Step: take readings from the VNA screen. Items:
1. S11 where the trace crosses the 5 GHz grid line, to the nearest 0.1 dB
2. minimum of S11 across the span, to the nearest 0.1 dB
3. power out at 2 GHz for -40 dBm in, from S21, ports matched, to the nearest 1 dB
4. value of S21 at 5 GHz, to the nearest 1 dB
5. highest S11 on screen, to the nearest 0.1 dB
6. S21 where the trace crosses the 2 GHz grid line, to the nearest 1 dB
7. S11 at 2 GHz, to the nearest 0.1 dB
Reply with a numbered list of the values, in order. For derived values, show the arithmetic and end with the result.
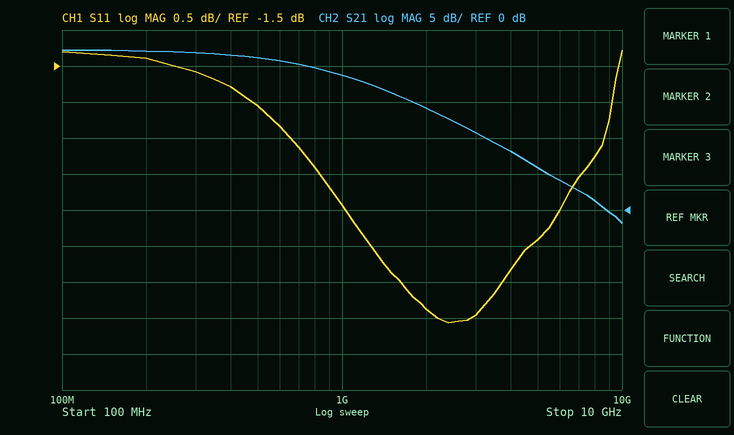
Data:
1. -3.9 dB
2. -5.1 dB
3. -40 dBm + (14 dB) = -26 dBm
4. 6 dB
5. -1.3 dB
6. 14 dB
7. -4.9 dB
